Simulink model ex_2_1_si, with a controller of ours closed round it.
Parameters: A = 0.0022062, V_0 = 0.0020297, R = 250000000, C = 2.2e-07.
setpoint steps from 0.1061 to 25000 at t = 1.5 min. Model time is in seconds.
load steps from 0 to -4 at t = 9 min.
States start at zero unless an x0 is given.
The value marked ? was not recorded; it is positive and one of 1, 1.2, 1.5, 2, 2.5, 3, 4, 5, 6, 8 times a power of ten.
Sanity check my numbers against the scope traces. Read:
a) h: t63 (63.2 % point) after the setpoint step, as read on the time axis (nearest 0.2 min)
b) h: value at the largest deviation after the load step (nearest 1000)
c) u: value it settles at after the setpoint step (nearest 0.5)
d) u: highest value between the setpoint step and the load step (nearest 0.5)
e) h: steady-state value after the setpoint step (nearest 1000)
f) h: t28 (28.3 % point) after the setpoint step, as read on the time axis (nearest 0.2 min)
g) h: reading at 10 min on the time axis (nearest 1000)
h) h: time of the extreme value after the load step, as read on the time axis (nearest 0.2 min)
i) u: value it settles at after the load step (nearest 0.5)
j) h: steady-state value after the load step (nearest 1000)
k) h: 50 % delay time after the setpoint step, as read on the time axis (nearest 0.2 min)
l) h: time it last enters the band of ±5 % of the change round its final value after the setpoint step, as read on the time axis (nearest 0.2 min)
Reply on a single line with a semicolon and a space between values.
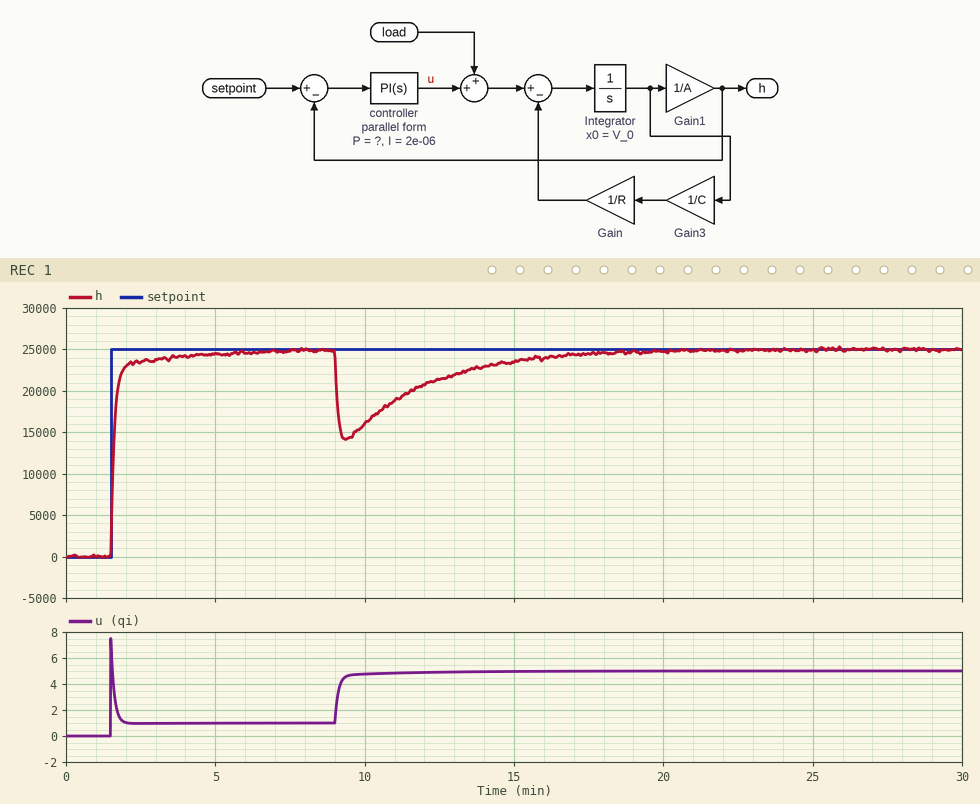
1.6 min; 14000; 1.0; 7.5; 25000; 1.6 min; 16000; 9.4 min; 5.0; 25000; 1.6 min; 3.0 min
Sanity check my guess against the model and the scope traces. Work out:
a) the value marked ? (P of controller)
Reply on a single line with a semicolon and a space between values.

0.0003
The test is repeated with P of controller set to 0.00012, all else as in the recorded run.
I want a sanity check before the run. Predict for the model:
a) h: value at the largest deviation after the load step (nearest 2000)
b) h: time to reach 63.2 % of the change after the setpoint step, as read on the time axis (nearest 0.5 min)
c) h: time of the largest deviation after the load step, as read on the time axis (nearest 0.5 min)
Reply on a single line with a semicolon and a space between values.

6000; 2.0 min; 9.5 min
